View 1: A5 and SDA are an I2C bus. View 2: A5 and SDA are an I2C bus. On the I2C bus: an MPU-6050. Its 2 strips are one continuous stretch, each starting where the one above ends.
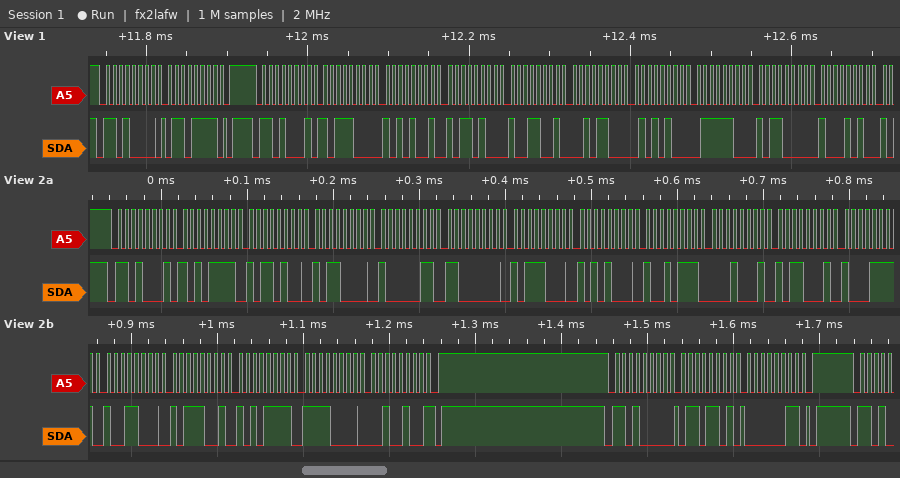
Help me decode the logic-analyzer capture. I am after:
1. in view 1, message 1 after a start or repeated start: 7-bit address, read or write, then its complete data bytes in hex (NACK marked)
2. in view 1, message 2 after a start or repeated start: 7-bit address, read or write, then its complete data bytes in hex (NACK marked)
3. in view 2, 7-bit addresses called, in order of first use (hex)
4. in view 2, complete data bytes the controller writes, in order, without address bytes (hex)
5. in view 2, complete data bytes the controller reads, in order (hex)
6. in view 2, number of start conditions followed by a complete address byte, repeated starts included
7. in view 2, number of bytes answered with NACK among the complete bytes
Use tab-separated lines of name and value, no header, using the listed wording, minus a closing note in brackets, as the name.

in view 1, message 1 after a start or repeated start: 7-bit address, read or write, then its complete data bytes in hex	0x68 write: 6F
in view 1, message 2 after a start or repeated start: 7-bit address, read or write, then its complete data bytes in hex	0x68 read: B8 A9 B4 99 2C 54 7C B0 8A
in view 2, 7-bit addresses called, in order of first use	0x68
in view 2, complete data bytes the controller writes, in order, without address bytes	6D 03
in view 2, complete data bytes the controller reads, in order	AF B4 B0 83 C0 B8 A8 97 11 B1 8F 98 B9 AF F0 24
in view 2, number of start conditions followed by a complete address byte, repeated starts included	2
in view 2, number of bytes answered with NACK among the complete bytes	1
